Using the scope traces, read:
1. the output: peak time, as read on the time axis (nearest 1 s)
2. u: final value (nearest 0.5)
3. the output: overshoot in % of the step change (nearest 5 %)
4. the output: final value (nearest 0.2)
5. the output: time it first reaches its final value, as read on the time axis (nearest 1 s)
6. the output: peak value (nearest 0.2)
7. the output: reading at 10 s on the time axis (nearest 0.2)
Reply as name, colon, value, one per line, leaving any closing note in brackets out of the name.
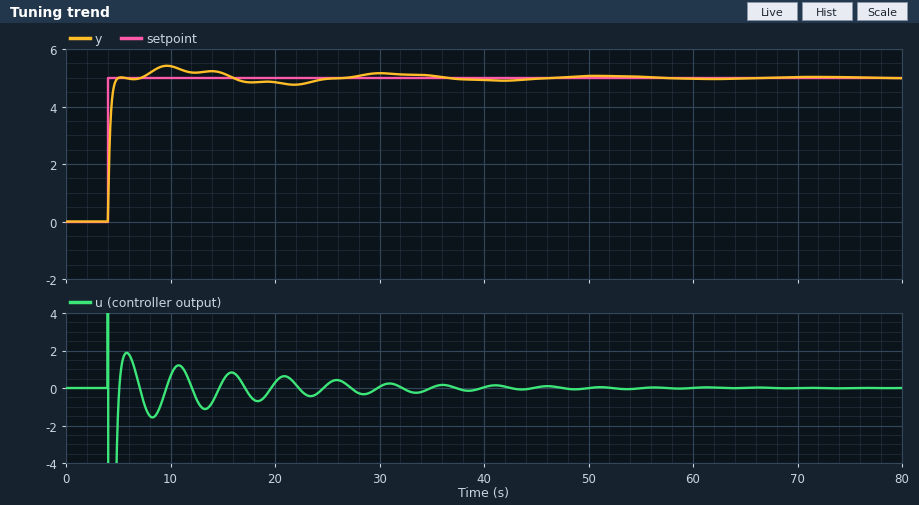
the output: peak time, as read on the time axis: 10 s
u: final value: 0.0
the output: overshoot in % of the step change: 10 %
the output: final value: 5.0
the output: time it first reaches its final value, as read on the time axis: 5 s
the output: peak value: 5.4
the output: reading at 10 s on the time axis: 5.4
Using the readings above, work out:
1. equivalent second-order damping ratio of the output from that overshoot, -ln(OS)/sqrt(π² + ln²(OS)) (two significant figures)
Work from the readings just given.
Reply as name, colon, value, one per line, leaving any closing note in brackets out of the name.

equivalent second-order damping ratio of the output from that overshoot, -ln(OS)/sqrt(π² + ln²(OS)): 0.59
